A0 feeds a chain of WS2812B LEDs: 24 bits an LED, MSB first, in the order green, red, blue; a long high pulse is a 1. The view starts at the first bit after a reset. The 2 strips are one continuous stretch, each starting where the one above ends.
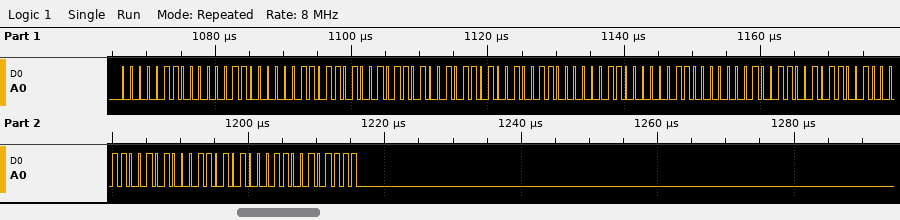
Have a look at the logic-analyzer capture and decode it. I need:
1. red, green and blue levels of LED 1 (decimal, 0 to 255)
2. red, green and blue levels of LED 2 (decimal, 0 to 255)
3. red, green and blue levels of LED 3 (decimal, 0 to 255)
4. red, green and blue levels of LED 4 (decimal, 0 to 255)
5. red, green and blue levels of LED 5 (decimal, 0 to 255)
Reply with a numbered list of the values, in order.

1. 6, 6, 6
2. 210, 210, 210
3. 96, 96, 96
4. 89, 38, 25
5. 163, 70, 47
